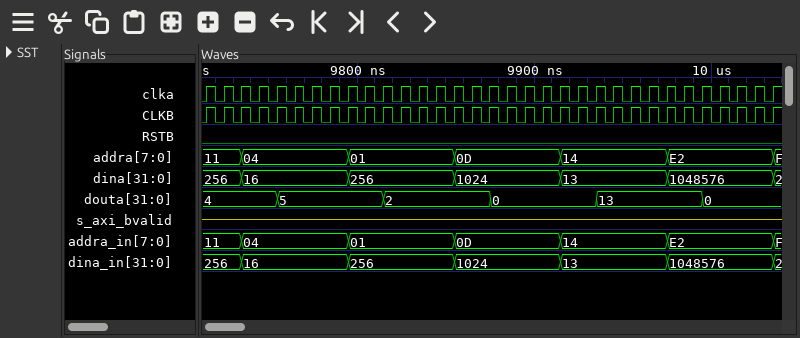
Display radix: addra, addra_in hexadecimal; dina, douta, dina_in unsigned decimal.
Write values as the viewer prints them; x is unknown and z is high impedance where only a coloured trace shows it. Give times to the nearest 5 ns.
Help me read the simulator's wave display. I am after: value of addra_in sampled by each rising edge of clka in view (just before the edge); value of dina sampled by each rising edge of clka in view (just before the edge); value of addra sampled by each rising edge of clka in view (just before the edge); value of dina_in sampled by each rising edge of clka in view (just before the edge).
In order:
11, 11, 11, 04, 04, 04, 04, 04, 04, 01, 01, 01, 01, 01, 01, 0D, 0D, 0D, 0D, 0D, 0D, 14, 14, 14, 14, 14, 14, E2, E2, E2, E2, E2, E2
256, 256, 256, 16, 16, 16, 16, 16, 16, 256, 256, 256, 256, 256, 256, 1024, 1024, 1024, 1024, 1024, 1024, 13, 13, 13, 13, 13, 13, 1048576, 1048576, 1048576, 1048576, 1048576, 1048576
11, 11, 11, 04, 04, 04, 04, 04, 04, 01, 01, 01, 01, 01, 01, 0D, 0D, 0D, 0D, 0D, 0D, 14, 14, 14, 14, 14, 14, E2, E2, E2, E2, E2, E2
256, 256, 256, 16, 16, 16, 16, 16, 16, 256, 256, 256, 256, 256, 256, 1024, 1024, 1024, 1024, 1024, 1024, 13, 13, 13, 13, 13, 13, 1048576, 1048576, 1048576, 1048576, 1048576, 1048576
